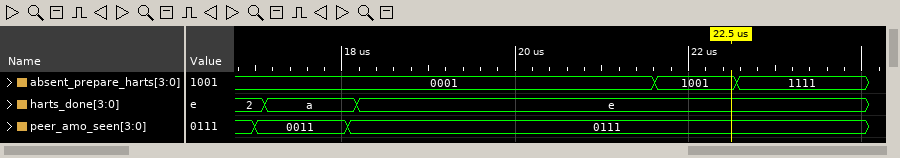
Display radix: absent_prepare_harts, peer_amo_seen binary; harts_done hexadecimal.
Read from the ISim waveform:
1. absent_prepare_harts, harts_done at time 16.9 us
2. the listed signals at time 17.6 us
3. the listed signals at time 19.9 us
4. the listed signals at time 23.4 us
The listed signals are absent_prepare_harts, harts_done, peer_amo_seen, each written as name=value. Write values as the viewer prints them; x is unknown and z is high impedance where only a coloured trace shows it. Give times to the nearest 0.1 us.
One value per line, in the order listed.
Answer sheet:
absent_prepare_harts=0001, harts_done=2
absent_prepare_harts=0001, harts_done=a, peer_amo_seen=0011
absent_prepare_harts=0001, harts_done=e, peer_amo_seen=0111
absent_prepare_harts=1111, harts_done=e, peer_amo_seen=0111
